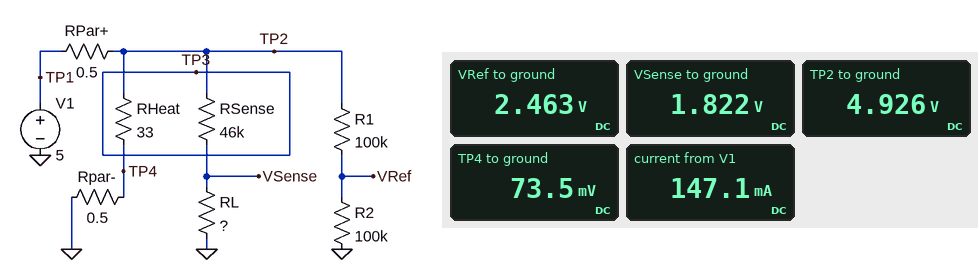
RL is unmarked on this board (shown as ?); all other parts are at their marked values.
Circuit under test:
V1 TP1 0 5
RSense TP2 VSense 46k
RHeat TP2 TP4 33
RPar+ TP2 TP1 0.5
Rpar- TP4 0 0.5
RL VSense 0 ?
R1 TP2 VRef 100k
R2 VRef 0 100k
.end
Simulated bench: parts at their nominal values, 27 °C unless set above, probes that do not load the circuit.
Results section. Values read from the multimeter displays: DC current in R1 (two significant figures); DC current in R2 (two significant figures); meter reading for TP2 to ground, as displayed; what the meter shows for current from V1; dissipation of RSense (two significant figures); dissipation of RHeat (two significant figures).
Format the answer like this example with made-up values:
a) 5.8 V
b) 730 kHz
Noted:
a) 25 µA
b) 25 µA
c) 4.926 V
d) 147.1 mA
e) 210 µW
f) 710 mW
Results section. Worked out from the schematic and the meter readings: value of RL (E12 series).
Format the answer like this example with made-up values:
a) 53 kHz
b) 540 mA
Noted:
a) 27 kΩ
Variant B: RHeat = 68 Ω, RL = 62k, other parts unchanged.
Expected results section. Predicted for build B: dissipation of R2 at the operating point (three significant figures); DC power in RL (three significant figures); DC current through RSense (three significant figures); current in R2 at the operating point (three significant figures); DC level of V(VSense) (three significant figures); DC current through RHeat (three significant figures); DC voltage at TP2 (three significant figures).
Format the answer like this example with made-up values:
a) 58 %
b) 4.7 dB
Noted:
a) 61.6 µW
b) 131 µW
c) 46.0 µA
d) 24.8 µA
e) 2.85 V
f) 72.5 mA
g) 4.96 V
